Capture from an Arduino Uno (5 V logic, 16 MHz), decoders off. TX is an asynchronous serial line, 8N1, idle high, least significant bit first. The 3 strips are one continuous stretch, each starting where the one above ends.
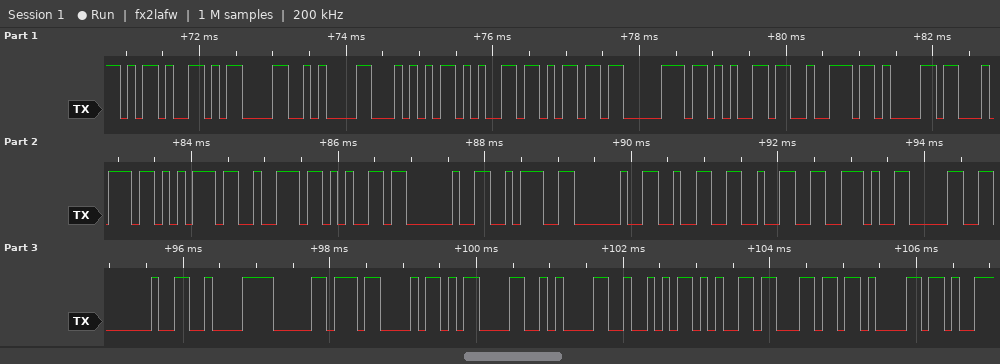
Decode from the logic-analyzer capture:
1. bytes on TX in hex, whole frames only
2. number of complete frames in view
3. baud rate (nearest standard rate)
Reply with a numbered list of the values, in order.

1. 2D 0D 0A 54 65 6D 70 65 72 61 74 75 72 65 20 3A 20 32 32 2E 30 20 C2 B0 43 0D 0A 52 65 6C 61
2. 31
3. 9600 baud
